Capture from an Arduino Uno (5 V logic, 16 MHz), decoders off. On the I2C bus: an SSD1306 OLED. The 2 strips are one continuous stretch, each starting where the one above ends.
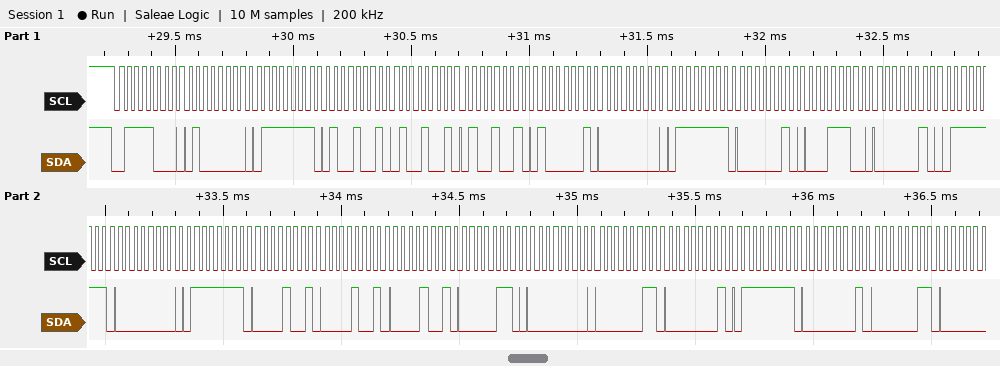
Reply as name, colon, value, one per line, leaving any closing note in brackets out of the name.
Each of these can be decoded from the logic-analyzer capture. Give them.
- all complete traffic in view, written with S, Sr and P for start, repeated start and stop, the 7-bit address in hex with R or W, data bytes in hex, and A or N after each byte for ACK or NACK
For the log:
all complete traffic in view, written with S, Sr and P for start, repeated start and stop, the 7-bit address in hex with R or W, data bytes in hex, and A or N after each byte for ACK or NACK: S 3CW A 40 A 7F A 49 A 49 A 49 A 41 A 00 A 7F A 02 A 1C A 02 A 7F A 00 A 7F A 09 A 09 A 09 A 06 A 00 A 03 A 01 A 7F A 01 A 03 A
